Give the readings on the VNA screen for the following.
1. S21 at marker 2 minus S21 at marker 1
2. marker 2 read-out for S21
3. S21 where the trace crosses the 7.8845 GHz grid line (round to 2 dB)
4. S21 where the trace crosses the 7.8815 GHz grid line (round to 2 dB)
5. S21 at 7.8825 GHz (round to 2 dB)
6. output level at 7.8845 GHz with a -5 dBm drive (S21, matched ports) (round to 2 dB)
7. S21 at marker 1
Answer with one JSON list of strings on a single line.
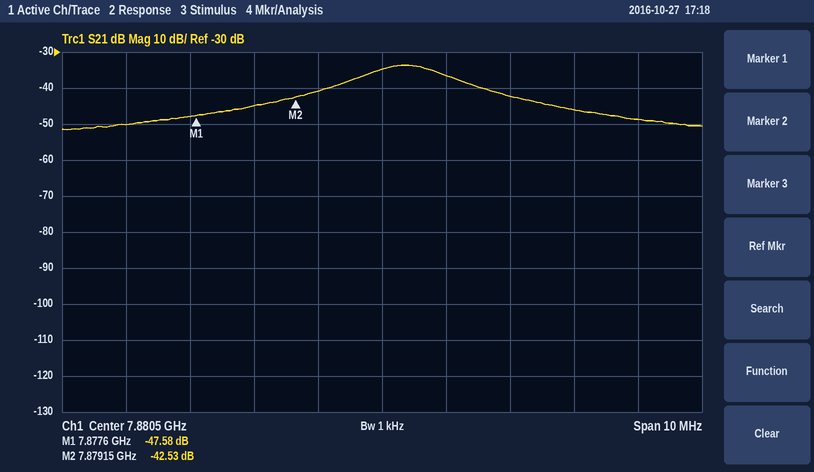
["5.05 dB", "-42.53 dB", "-48 dB", "-36 dB", "-42 dB", "-54 dBm", "-47.58 dB"]
